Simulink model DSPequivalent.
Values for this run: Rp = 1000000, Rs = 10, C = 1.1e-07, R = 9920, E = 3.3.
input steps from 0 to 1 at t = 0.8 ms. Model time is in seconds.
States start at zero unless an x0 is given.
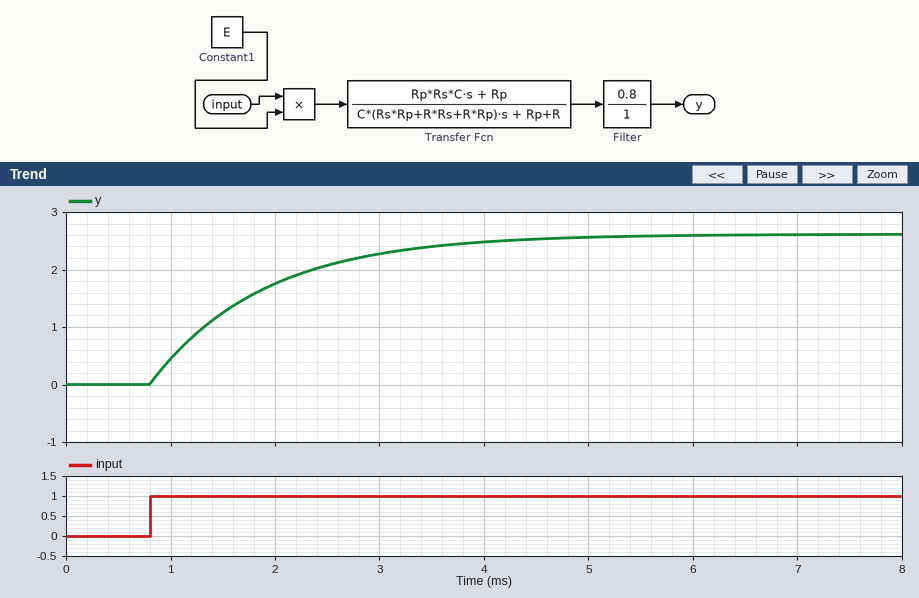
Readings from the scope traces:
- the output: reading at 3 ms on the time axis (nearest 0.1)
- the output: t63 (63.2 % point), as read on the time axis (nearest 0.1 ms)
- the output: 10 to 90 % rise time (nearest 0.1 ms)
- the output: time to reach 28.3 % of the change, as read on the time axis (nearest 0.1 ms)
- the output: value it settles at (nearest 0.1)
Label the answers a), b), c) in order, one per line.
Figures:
a) 2.3
b) 1.9 ms
c) 2.4 ms
d) 1.2 ms
e) 2.6
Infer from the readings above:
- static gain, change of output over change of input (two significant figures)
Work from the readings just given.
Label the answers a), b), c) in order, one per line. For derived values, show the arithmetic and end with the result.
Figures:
a) (2.6 - 0) / (1 - 0) = 2.6
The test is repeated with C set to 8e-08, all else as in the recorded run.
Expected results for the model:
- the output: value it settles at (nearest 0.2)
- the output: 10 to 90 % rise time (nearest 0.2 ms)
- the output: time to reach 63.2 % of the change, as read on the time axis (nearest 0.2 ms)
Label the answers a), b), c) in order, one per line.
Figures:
a) 2.6
b) 1.8 ms
c) 1.6 ms
